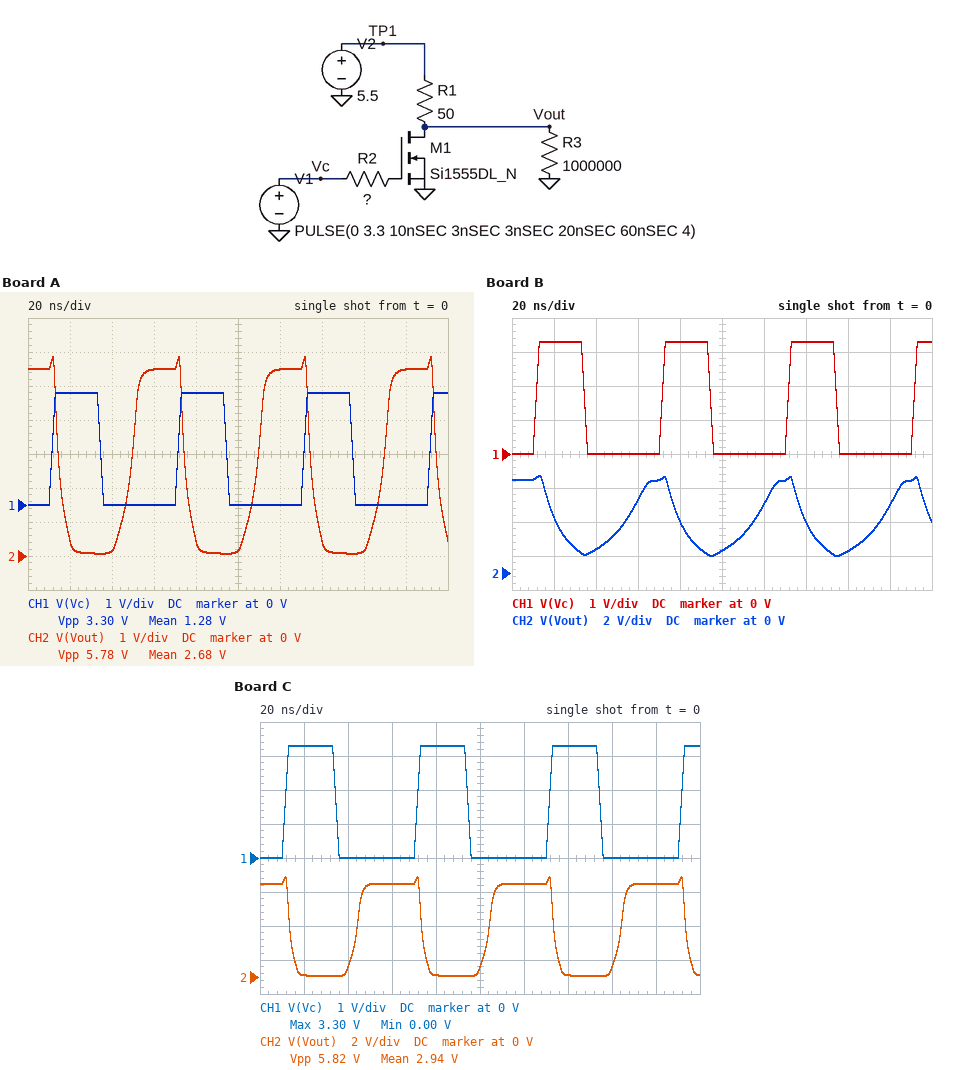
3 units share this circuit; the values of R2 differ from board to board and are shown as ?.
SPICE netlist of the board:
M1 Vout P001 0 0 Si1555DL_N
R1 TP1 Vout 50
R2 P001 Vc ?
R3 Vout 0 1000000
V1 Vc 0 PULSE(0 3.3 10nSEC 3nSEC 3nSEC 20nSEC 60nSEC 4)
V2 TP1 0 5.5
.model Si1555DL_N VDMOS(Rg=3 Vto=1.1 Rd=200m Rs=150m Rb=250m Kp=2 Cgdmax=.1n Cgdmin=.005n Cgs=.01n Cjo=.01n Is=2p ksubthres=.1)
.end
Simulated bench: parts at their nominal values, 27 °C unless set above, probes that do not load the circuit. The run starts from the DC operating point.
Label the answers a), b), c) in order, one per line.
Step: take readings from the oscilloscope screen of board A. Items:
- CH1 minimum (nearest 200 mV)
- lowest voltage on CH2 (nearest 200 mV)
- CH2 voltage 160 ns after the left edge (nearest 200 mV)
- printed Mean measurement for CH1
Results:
a) 0 V
b) 0 V
c) 200 mV
d) 1.28 V
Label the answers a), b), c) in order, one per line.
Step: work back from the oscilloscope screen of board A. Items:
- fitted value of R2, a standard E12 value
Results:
a) 68 Ω
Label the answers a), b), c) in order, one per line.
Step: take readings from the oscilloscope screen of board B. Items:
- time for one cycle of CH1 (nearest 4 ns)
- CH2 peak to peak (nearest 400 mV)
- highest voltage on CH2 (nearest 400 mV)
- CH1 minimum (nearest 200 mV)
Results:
a) 60 ns
b) 4.8 V
c) 5.6 V
d) 0 V
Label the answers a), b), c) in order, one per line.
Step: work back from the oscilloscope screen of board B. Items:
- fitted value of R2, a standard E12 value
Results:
a) 270 Ω
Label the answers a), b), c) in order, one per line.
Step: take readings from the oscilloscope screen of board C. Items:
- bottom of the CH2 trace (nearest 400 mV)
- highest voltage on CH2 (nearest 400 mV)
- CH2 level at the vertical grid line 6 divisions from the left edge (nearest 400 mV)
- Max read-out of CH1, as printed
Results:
a) 0 V
b) 6.0 V
c) 5.6 V
d) 3.30 V
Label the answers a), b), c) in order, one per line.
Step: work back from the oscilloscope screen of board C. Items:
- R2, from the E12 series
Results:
a) 39 Ω
